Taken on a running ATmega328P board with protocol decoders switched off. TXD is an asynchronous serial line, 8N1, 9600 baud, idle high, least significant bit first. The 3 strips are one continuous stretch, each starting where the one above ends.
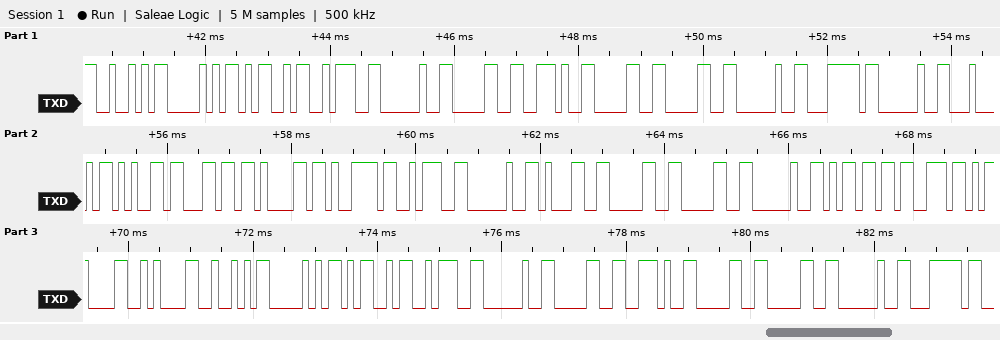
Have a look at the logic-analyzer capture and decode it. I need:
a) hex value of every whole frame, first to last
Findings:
52 50 4D 3A 20 30 2E 30 30 20 7C 20 44 65 6C 61 79 3A 20 31 30 30 20 6D 73 0D 0A 52 50 4D 3A 20 30 2E 30 30 20 7C
